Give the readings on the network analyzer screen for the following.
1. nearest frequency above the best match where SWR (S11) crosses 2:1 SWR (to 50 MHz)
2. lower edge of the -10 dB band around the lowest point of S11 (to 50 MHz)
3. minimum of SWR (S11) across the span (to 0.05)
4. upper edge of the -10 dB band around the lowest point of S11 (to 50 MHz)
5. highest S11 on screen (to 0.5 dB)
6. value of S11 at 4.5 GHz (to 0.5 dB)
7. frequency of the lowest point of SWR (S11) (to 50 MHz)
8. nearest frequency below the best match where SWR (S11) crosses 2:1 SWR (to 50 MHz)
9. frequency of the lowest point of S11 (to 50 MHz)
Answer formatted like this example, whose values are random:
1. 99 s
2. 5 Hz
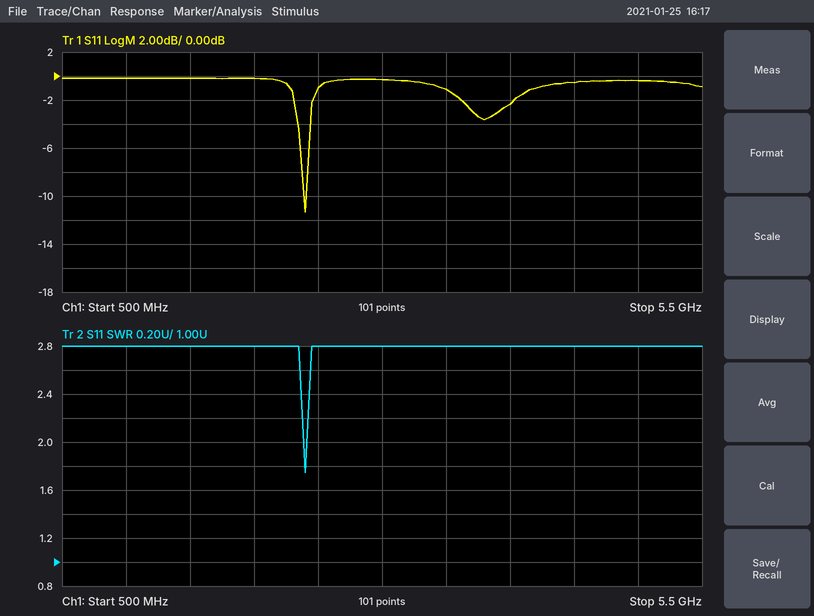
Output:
1. 2.40 GHz
2. 2.40 GHz
3. 1.75
4. 2.40 GHz
5. 0.0 dB
6. -0.5 dB
7. 2.40 GHz
8. 2.40 GHz
9. 2.40 GHz
